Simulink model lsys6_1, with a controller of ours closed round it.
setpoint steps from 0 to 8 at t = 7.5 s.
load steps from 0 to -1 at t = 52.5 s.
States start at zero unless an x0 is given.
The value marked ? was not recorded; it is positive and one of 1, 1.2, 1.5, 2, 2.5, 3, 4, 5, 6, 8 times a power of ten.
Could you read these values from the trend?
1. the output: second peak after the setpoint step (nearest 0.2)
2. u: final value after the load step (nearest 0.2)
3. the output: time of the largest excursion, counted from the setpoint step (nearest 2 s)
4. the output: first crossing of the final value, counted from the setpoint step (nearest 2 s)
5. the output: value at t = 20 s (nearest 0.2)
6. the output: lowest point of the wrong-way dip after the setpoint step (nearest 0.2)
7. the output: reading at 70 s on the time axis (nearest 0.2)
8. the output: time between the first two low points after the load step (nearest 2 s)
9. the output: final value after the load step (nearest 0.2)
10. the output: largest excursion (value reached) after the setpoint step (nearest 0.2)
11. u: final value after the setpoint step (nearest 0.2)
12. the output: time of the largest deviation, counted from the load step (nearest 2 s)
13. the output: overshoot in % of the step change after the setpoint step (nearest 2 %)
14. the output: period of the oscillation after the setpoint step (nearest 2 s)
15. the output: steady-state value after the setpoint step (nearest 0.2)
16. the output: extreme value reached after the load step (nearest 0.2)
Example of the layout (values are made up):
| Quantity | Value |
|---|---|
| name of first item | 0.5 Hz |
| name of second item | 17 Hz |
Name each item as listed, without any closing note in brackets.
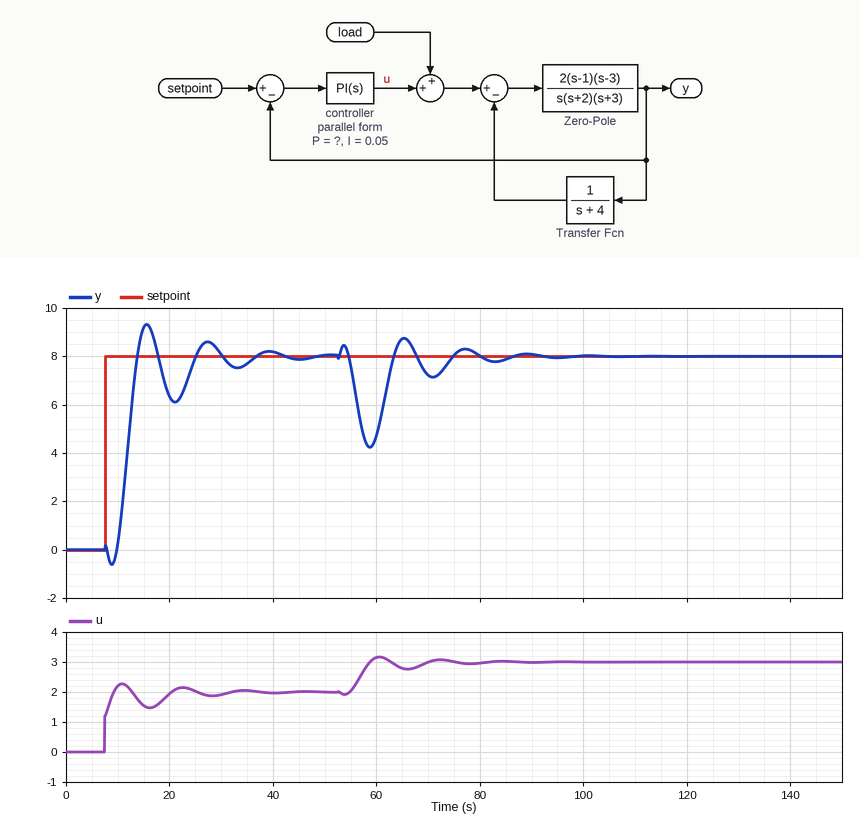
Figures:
| Quantity | Value |
|---|---|
| the output: second peak after the setpoint step | 8.6 |
| u: final value after the load step | 3.0 |
| the output: time of the largest excursion, counted from the setpoint step | 8 s |
| the output: first crossing of the final value, counted from the setpoint step | 6 s |
| the output: value at t = 20 s | 6.4 |
| the output: lowest point of the wrong-way dip after the setpoint step | -0.6 |
| the output: reading at 70 s on the time axis | 7.2 |
| the output: time between the first two low points after the load step | 12 s |
| the output: final value after the load step | 8.0 |
| the output: largest excursion (value reached) after the setpoint step | 9.4 |
| u: final value after the setpoint step | 2.0 |
| the output: time of the largest deviation, counted from the load step | 6 s |
| the output: overshoot in % of the step change after the setpoint step | 16 % |
| the output: period of the oscillation after the setpoint step | 12 s |
| the output: steady-state value after the setpoint step | 8.0 |
| the output: extreme value reached after the load step | 4.2 |
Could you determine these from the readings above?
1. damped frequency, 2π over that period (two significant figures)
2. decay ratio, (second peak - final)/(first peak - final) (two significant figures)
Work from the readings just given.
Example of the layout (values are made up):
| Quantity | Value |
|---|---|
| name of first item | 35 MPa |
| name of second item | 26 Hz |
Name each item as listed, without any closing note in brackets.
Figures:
| Quantity | Value |
|---|---|
| damped frequency, 2π over that period | 0.52 rad/s |
| decay ratio, (second peak - final)/(first peak - final) | 0.43 |
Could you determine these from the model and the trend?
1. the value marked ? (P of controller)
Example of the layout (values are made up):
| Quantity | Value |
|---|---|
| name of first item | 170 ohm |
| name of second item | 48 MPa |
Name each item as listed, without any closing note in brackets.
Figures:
| Quantity | Value |
|---|---|
| the value marked ? | 0.15 |
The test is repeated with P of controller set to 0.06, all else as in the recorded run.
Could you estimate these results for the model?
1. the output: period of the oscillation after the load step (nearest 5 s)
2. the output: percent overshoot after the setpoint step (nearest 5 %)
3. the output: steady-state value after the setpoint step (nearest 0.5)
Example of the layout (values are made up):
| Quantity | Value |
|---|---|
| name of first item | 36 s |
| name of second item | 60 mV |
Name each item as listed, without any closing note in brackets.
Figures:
| Quantity | Value |
|---|---|
| the output: period of the oscillation after the load step | 15 s |
| the output: percent overshoot after the setpoint step | 20 % |
| the output: steady-state value after the setpoint step | 8.0 |
